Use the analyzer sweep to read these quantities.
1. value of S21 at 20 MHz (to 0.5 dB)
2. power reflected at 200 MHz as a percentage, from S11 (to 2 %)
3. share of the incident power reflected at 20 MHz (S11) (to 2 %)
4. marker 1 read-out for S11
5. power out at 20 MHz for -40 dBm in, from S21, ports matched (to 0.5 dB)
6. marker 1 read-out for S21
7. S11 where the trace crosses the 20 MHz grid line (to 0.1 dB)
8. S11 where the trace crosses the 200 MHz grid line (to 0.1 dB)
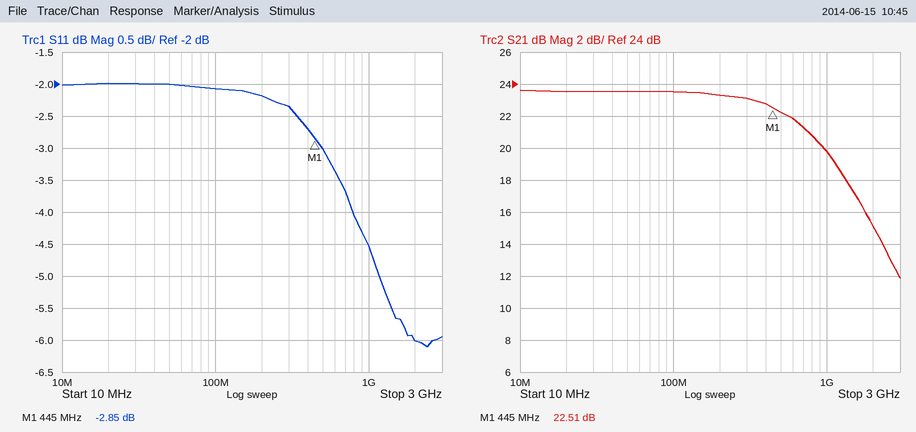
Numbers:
23.5 dB
60 %
64 %
-2.85 dB
-16.5 dBm
22.51 dB
-2.0 dB
-2.2 dB
